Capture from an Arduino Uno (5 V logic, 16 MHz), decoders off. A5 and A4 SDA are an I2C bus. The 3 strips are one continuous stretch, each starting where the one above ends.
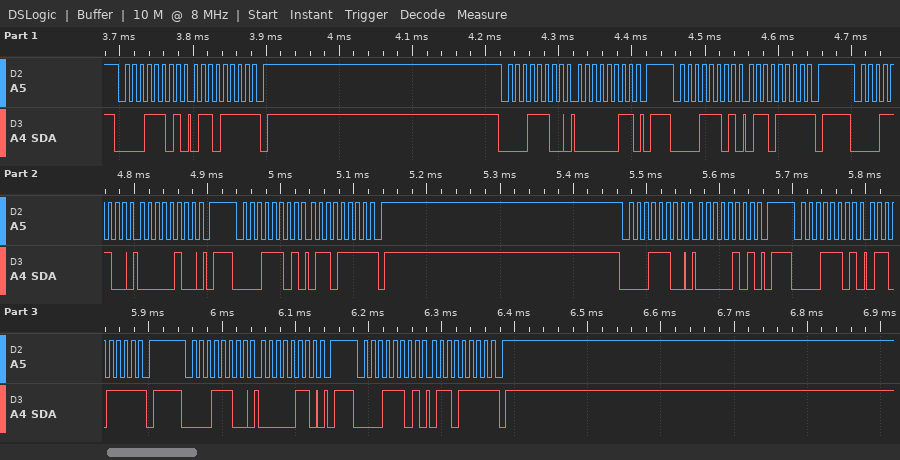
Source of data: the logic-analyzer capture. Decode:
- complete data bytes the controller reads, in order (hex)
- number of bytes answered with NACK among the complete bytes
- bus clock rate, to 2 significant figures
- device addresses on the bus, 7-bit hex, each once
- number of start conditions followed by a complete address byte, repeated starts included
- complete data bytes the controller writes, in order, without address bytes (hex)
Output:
6F 6F 6F 6F 6F
5
100 kHz
0x0E
9
03 04 05 06
